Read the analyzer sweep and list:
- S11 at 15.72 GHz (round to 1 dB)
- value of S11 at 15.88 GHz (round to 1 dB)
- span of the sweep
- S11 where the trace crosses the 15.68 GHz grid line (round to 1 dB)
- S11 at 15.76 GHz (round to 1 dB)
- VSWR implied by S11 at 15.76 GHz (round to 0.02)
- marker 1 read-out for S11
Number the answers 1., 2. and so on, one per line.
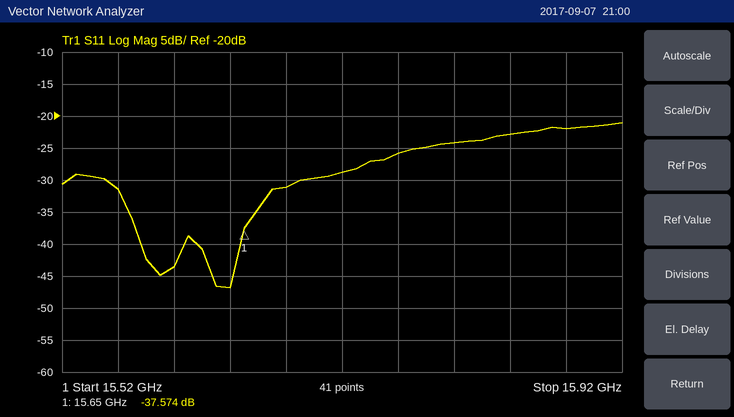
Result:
1. -29 dB
2. -22 dB
3. 400 MHz
4. -31 dB
5. -26 dB
6. 1.10
7. -37.574 dB
